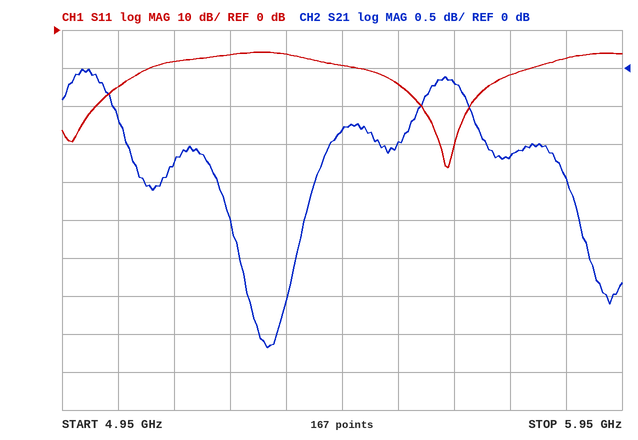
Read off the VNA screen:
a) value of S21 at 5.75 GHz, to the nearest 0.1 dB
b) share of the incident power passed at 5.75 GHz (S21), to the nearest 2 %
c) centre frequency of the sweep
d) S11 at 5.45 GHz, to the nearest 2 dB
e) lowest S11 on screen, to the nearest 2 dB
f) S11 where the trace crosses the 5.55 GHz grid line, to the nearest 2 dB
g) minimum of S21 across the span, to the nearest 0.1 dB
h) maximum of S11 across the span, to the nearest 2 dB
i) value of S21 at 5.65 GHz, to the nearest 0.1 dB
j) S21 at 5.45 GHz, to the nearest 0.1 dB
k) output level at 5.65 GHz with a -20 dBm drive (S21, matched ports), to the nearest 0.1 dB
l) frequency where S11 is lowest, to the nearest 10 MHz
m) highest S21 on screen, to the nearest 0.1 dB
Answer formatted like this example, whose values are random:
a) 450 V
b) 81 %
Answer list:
a) -1.2 dB
b) 76 %
c) 5.45 GHz
d) -10 dB
e) -36 dB
f) -14 dB
g) -3.7 dB
h) -6 dB
i) -0.2 dB
j) -0.8 dB
k) -20.2 dBm
l) 5.64 GHz
m) 0.0 dB
